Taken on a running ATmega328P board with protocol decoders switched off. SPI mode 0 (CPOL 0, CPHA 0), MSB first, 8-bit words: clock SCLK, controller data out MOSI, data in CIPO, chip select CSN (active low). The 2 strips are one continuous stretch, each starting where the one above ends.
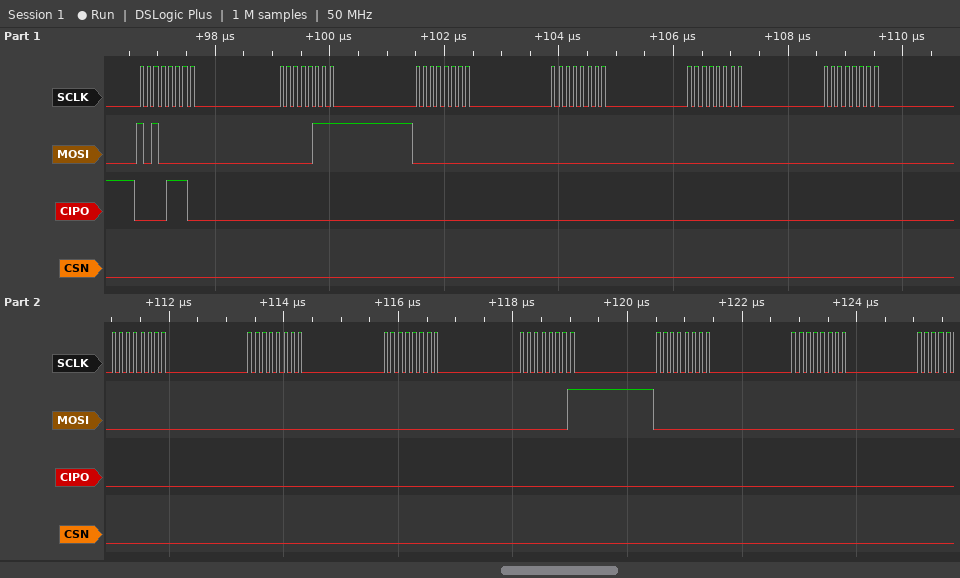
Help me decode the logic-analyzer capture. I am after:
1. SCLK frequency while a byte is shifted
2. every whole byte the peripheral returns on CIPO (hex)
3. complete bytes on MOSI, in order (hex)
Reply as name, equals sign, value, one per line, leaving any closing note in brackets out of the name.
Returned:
SCLK frequency while a byte is shifted = 8 MHz
every whole byte the peripheral returns on CIPO = 0E 00 00 00 00 00 00 00 00 00 00 00
complete bytes on MOSI, in order = A0 07 00 00 00 00 00 00 00 01 00 00
